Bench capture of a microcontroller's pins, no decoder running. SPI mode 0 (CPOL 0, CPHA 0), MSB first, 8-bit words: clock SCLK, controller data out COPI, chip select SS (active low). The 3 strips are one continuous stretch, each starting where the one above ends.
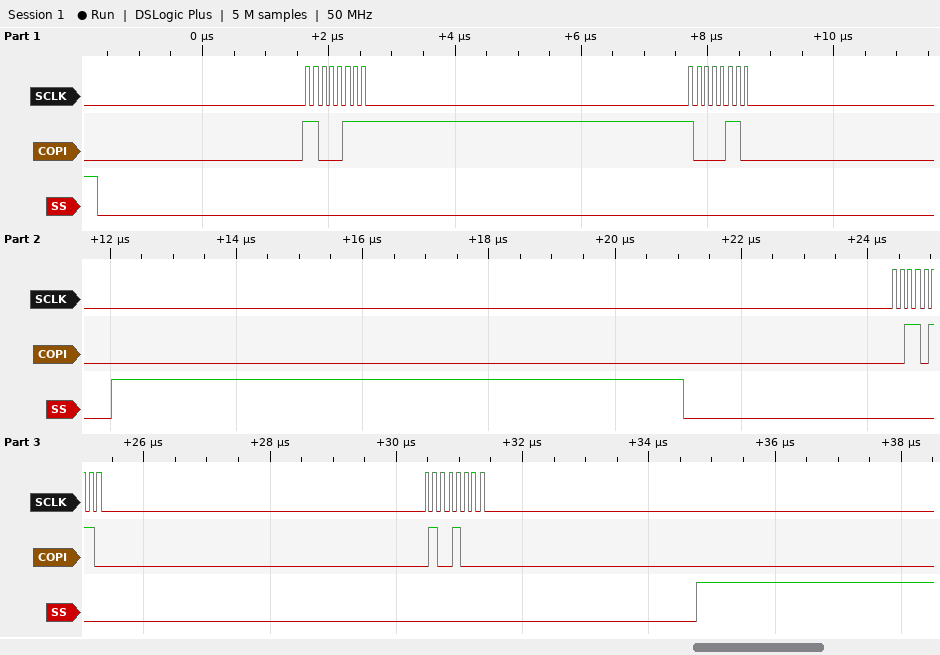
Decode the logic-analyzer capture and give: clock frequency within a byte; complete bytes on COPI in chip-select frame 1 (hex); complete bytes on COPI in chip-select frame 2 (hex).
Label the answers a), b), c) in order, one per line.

a) 8 MHz
b) C7 86
c) 36 48
